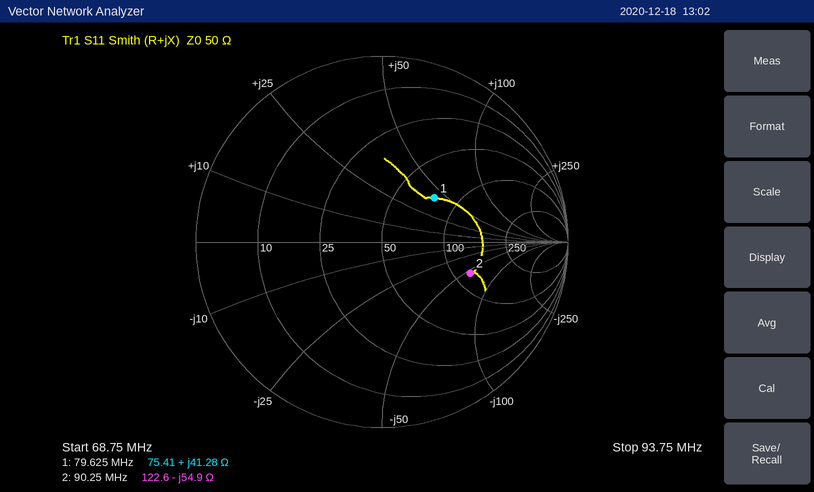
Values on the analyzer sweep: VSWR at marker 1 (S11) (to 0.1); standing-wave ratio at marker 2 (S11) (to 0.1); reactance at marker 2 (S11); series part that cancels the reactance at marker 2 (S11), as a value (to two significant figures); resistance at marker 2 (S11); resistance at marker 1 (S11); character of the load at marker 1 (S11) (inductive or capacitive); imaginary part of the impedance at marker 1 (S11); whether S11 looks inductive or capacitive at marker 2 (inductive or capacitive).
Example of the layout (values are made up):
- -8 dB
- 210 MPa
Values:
- 2.2
- 3.0
- -54.9 Ω
- 97 nH
- 122.6 Ω
- 75.41 Ω
- inductive
- +41.28 Ω
- capacitive
